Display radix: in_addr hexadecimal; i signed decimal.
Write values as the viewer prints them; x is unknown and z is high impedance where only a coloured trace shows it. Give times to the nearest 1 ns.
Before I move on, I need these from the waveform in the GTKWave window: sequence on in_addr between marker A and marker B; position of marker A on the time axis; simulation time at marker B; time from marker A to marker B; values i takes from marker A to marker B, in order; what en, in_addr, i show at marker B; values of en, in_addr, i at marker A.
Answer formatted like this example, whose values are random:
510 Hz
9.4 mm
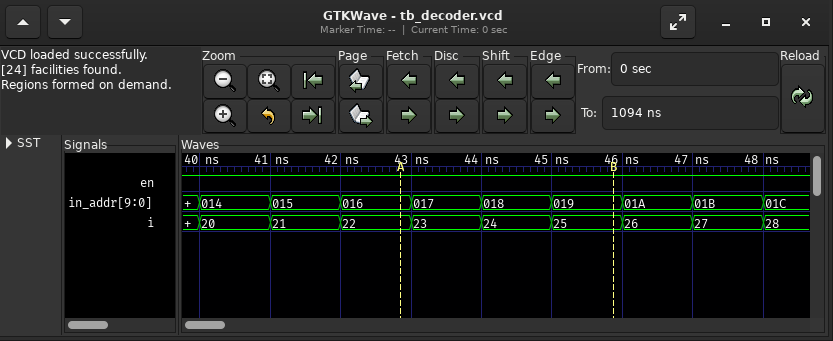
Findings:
016, 017, 018, 019
43 ns
46 ns
3 ns
22, 23, 24, 25
en=1, in_addr=019, i=25
en=1, in_addr=016, i=22
